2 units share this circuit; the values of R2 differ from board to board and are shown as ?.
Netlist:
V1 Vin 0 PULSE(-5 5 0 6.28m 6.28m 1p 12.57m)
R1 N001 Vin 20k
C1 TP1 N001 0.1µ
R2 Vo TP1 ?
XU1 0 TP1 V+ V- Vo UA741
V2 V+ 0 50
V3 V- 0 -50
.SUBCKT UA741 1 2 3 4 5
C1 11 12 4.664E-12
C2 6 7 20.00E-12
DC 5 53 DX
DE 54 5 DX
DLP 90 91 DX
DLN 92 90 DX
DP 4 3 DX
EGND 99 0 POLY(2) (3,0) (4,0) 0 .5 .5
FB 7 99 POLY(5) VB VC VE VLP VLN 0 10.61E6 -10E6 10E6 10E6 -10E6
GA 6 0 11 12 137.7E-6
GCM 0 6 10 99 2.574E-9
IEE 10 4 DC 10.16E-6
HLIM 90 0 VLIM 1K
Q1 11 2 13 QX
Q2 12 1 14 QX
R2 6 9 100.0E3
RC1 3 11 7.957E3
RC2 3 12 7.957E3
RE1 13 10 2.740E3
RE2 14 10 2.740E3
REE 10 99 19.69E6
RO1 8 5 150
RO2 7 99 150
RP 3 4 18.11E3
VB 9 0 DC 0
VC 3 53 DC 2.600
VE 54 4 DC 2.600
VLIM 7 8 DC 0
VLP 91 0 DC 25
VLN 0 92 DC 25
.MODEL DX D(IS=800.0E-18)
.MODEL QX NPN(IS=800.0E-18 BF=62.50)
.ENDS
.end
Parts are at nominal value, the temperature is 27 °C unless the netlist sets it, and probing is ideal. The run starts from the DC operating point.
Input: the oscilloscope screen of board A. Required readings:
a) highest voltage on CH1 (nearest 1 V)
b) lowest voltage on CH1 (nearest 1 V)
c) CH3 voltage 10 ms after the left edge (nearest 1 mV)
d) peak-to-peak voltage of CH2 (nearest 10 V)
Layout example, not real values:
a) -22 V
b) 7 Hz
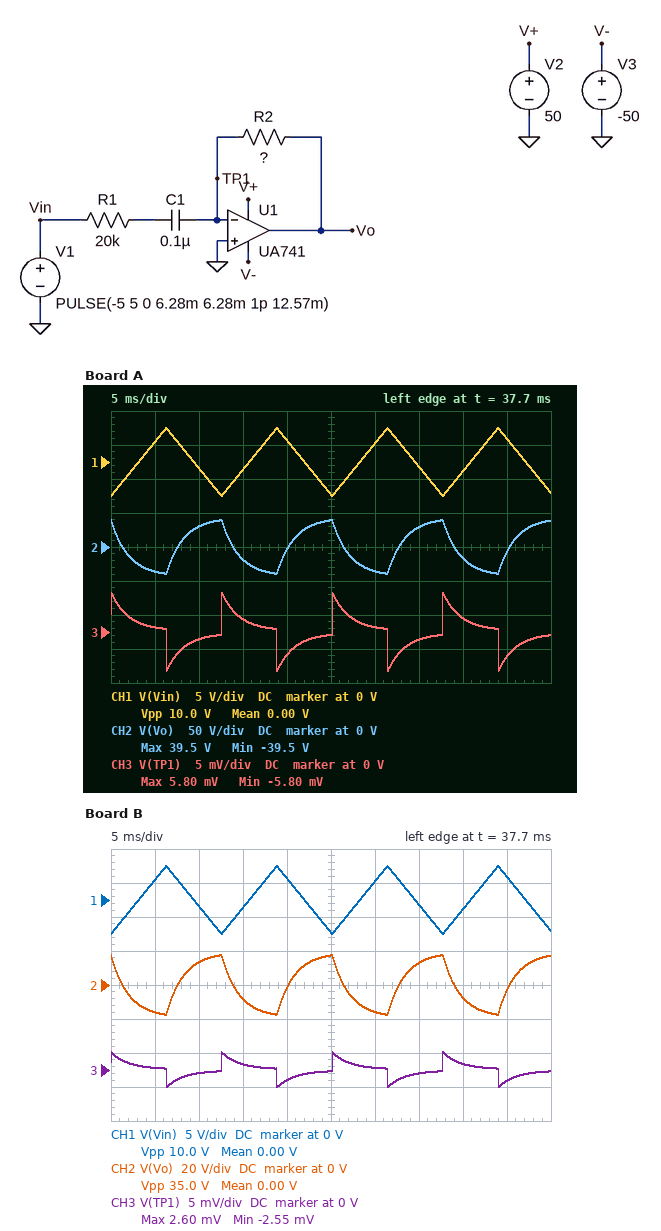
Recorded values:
a) 5 V
b) -5 V
c) -1 mV
d) 80 V
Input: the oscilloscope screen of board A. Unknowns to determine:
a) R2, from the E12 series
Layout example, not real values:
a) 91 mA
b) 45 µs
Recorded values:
a) 270 kΩ
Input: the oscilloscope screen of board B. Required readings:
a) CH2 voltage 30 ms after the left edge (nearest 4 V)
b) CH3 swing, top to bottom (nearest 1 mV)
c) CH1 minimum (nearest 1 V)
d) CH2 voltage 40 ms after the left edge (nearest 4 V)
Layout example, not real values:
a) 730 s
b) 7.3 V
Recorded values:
a) -16 V
b) 5 mV
c) -5 V
d) -8 V
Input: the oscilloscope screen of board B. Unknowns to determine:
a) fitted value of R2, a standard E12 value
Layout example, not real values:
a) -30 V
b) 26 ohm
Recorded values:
a) 120 kΩ
